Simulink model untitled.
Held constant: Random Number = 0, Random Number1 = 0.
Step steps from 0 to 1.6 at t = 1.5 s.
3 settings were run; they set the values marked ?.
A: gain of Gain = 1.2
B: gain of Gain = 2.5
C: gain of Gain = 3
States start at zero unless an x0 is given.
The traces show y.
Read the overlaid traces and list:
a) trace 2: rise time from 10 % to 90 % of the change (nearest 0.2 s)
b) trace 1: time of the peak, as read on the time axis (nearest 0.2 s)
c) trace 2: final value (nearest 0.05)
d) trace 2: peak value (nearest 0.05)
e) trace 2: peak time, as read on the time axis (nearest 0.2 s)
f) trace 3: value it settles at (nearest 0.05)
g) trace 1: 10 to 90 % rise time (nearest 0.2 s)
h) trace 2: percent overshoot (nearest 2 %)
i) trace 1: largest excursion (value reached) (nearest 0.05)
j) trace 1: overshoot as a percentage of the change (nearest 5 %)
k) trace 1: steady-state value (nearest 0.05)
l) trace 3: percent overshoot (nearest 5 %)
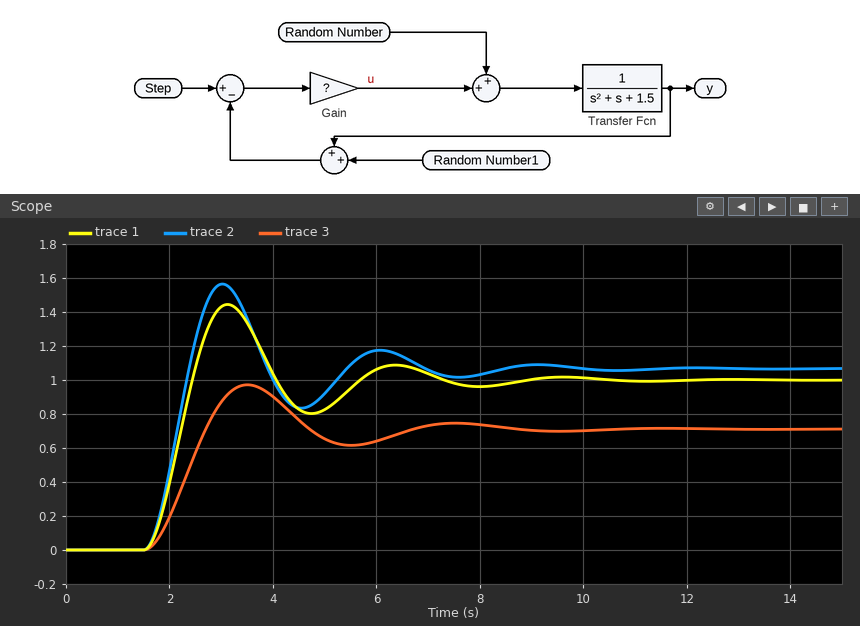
0.6 s
3.2 s
1.05
1.55
3.0 s
0.70
0.6 s
46 %
1.45
45 %
1.00
35 %
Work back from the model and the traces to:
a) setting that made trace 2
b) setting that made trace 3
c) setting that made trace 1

C
A
B
